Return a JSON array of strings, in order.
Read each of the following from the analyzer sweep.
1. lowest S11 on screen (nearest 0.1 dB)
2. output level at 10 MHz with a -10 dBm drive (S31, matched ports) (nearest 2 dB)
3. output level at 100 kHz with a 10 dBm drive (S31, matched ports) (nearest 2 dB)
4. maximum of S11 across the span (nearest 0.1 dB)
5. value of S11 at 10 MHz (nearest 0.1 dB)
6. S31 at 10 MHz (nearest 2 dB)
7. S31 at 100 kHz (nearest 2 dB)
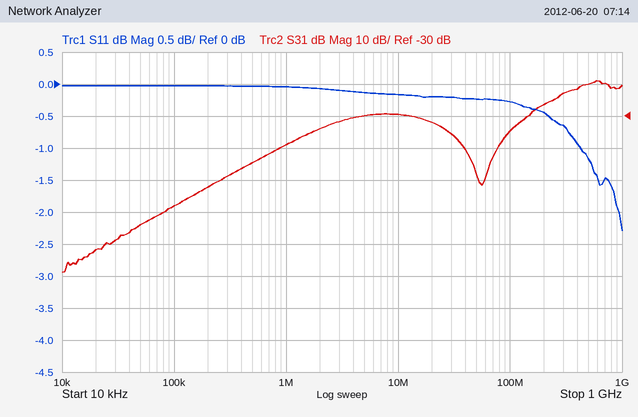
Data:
["-2.3 dB", "-40 dBm", "-48 dBm", "0.0 dB", "-0.2 dB", "-30 dB", "-58 dB"]
